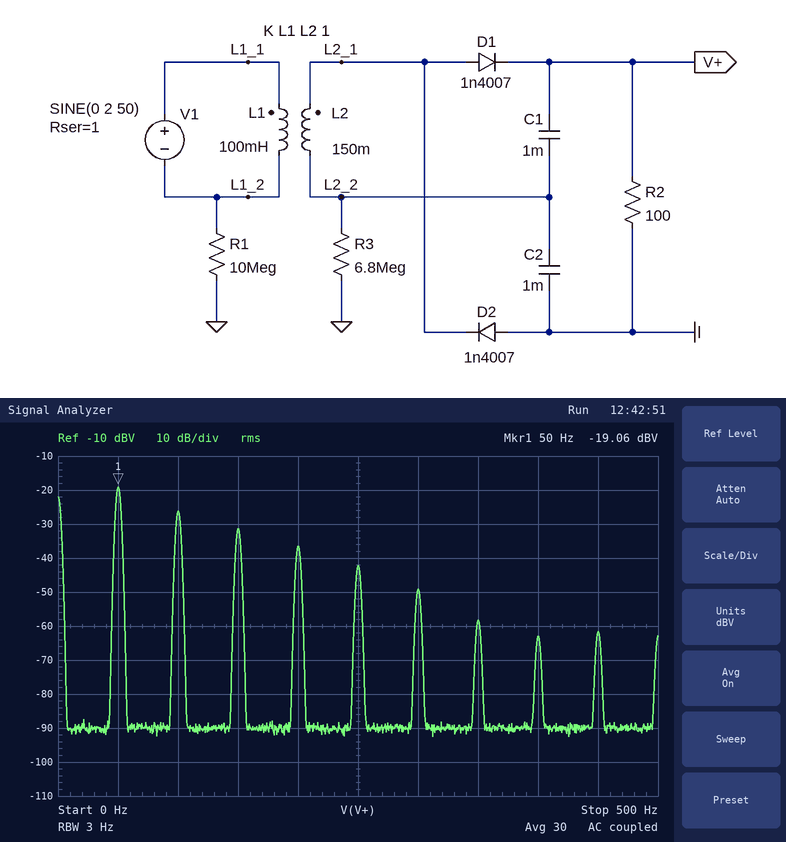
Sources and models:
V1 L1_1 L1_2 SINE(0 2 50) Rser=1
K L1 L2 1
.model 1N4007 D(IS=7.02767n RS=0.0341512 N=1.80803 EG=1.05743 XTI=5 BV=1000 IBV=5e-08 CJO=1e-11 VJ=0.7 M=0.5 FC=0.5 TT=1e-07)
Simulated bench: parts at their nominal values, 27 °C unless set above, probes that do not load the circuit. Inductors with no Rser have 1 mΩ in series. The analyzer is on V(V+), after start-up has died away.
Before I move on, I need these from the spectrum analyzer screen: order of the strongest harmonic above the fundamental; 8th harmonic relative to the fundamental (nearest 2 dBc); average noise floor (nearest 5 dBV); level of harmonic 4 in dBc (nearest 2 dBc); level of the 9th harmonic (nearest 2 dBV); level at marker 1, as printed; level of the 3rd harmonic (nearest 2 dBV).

2
-44 dBc
-90 dBV
-18 dBc
-62 dBV
-19.06 dBV
-32 dBV
